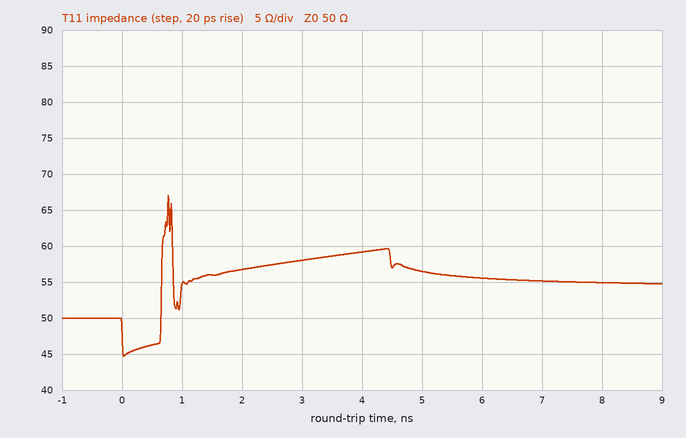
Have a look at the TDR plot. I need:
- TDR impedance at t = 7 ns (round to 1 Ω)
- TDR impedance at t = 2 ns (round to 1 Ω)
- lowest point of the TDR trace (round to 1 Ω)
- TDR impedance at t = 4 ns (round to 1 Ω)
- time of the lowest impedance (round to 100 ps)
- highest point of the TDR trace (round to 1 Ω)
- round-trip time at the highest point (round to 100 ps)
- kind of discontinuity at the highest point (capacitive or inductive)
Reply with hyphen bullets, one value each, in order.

- 55 Ω
- 57 Ω
- 45 Ω
- 59 Ω
- 0.0 ns
- 67 Ω
- 800 ps
- inductive
